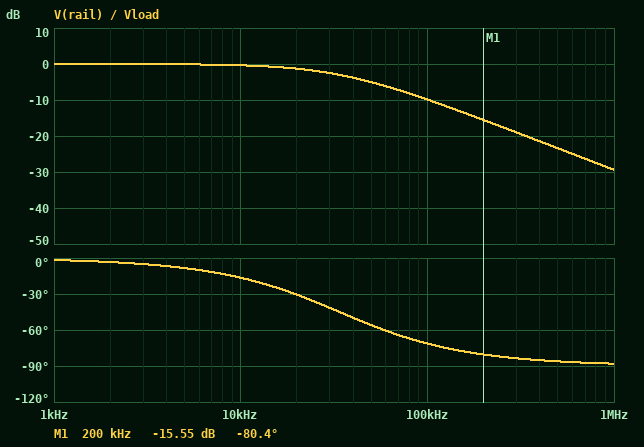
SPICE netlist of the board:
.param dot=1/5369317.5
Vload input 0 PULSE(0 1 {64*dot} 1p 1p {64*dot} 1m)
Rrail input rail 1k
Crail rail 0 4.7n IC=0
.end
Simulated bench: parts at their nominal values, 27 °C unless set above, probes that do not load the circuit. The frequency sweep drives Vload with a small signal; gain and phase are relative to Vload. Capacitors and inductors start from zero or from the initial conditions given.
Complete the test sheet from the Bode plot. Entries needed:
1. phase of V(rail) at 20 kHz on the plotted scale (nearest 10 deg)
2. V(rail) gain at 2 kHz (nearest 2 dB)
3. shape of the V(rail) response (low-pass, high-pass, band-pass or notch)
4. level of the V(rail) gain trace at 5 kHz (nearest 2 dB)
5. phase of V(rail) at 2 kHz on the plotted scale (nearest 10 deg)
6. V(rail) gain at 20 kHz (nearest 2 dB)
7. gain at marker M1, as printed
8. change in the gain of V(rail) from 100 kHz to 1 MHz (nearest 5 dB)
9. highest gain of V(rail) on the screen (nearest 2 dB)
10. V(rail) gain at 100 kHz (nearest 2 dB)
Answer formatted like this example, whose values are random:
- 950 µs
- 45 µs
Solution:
- -30 deg
- 0 dB
- low-pass
- 0 dB
- 0 deg
- -2 dB
- -15.55 dB
- -20 dB
- 0 dB
- -10 dB
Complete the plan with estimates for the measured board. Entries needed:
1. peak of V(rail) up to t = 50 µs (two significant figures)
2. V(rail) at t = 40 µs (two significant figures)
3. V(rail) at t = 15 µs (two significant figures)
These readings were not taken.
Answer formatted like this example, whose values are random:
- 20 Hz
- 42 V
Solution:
- 920 mV
- 30 mV
- 480 mV
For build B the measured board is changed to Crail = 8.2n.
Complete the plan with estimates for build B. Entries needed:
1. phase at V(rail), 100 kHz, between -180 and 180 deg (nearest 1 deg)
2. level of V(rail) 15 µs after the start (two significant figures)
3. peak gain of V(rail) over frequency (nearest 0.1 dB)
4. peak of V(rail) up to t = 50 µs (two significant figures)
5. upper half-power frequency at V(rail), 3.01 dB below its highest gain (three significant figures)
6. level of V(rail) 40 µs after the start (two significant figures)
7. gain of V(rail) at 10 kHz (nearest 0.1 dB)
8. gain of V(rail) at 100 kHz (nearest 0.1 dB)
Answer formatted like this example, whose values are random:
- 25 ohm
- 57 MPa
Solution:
- -79 deg
- 310 mV
- 0 dB
- 770 mV
- 19.4 kHz
- 110 mV
- -1.0 dB
- -14.4 dB
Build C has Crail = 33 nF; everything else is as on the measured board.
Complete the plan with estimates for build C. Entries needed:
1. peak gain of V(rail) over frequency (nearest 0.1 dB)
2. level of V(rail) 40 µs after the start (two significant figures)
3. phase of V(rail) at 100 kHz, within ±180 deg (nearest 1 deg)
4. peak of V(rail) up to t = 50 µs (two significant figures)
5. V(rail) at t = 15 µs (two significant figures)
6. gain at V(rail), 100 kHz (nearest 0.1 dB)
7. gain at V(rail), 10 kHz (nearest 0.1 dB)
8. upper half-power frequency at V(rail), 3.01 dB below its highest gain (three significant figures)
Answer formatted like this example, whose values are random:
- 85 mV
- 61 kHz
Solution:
- 0 dB
- 190 mV
- -87 deg
- 300 mV
- 89 mV
- -26.3 dB
- -7.2 dB
- 4.82 kHz
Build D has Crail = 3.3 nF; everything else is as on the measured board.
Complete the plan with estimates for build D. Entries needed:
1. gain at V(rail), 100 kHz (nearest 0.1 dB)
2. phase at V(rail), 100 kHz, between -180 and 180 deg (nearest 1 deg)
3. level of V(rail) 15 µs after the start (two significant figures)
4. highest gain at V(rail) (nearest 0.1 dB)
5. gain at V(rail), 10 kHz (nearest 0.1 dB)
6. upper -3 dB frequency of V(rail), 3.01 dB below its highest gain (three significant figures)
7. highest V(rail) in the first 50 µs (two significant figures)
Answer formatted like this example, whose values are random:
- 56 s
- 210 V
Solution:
- -7.2 dB
- -64 deg
- 610 mV
- 0 dB
- -0.2 dB
- 48.2 kHz
- 970 mV
